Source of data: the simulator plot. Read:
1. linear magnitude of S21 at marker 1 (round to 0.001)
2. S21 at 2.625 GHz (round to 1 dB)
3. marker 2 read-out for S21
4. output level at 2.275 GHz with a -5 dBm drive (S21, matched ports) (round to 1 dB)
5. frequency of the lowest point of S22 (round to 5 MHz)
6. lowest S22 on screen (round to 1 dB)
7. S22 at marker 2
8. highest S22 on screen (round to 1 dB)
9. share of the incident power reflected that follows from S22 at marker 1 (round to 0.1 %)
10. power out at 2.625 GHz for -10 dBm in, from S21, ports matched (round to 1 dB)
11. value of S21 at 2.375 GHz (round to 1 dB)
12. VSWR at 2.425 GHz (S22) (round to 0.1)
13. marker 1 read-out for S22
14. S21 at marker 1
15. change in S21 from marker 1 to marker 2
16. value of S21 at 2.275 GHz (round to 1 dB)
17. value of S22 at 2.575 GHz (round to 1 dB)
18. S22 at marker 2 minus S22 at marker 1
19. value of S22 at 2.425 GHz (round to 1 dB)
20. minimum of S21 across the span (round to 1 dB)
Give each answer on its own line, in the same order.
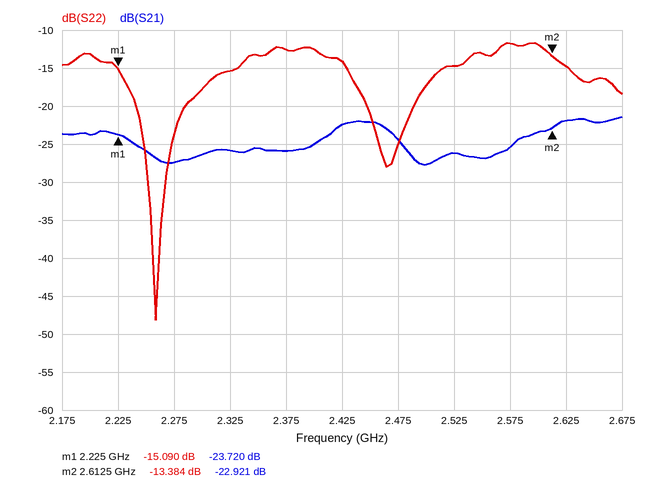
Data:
0.065
-22 dB
-22.921 dB
-32 dBm
2.260 GHz
-48 dB
-13.384 dB
-12 dB
3.1 %
-32 dBm
-26 dB
1.5
-15.090 dB
-23.720 dB
0.799 dB
-27 dB
-12 dB
1.706 dB
-14 dB
-28 dB
